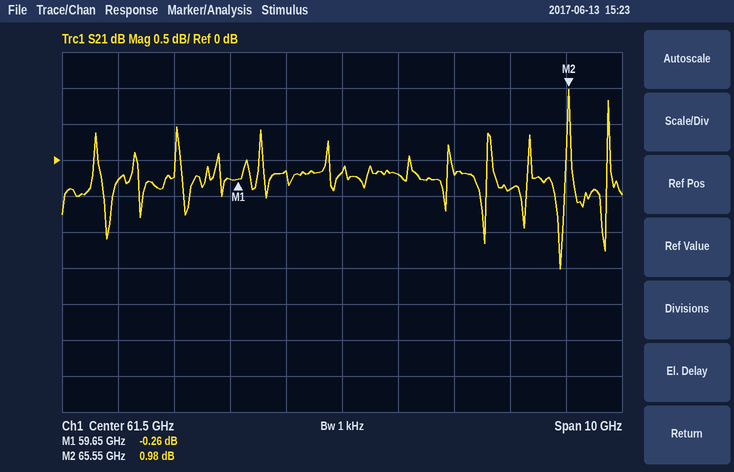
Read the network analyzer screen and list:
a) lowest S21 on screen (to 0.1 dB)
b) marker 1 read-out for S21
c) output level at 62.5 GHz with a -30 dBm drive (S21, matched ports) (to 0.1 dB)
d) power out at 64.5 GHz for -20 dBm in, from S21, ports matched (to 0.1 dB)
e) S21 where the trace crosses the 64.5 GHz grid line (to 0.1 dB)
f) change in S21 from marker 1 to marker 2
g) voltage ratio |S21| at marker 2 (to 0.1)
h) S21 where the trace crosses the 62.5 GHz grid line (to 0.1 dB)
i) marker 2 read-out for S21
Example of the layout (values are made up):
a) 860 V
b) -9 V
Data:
a) -1.5 dB
b) -0.26 dB
c) -30.2 dBm
d) -20.4 dBm
e) -0.4 dB
f) 1.24 dB
g) 1.1
h) -0.2 dB
i) 0.98 dB
